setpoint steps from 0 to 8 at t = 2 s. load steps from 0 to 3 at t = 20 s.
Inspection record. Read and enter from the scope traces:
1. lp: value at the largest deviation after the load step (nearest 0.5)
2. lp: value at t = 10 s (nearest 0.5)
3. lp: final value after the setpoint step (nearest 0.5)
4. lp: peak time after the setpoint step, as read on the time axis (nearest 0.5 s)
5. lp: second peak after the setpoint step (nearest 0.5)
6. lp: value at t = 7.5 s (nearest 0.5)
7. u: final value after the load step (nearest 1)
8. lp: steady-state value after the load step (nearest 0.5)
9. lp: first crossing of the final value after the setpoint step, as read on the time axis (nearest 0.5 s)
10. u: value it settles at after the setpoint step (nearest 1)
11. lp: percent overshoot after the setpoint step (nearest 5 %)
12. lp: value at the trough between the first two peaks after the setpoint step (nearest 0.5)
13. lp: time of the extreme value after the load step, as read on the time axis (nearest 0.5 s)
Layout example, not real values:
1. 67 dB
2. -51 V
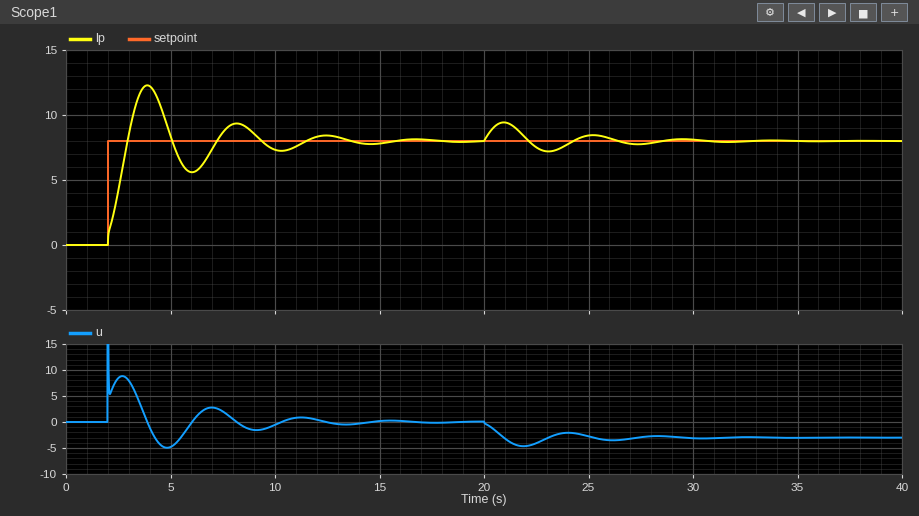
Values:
1. 9.5
2. 7.5
3. 8.0
4. 4.0 s
5. 9.5
6. 8.5
7. -3
8. 8.0
9. 3.0 s
10. 0
11. 55 %
12. 5.5
13. 21.0 s
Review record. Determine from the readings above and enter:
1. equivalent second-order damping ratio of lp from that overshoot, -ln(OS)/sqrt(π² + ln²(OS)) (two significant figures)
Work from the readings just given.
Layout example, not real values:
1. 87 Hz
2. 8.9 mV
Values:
1. 0.19
